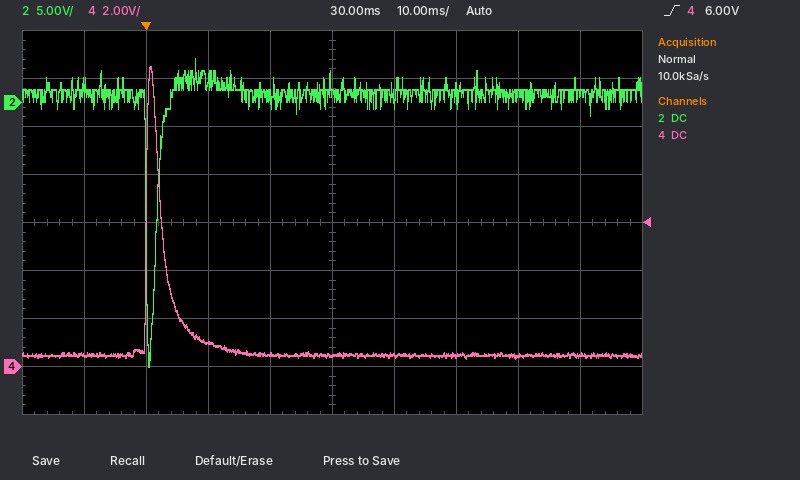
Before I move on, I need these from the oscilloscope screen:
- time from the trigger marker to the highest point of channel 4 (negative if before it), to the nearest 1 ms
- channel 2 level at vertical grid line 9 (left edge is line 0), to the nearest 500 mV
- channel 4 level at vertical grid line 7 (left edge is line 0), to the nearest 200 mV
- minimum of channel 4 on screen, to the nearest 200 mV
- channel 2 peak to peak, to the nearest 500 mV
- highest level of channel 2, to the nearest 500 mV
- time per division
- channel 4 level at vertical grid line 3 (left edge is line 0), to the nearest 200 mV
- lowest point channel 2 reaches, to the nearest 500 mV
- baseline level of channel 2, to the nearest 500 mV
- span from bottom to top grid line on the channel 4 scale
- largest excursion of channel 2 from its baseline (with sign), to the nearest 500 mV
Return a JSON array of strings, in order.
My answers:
["+1 ms", "1.0 V", "400 mV", "400 mV", "32.0 V", "4.5 V", "10 ms", "1.0 V", "-27.5 V", "1.0 V", "16 V", "-28.5 V"]
